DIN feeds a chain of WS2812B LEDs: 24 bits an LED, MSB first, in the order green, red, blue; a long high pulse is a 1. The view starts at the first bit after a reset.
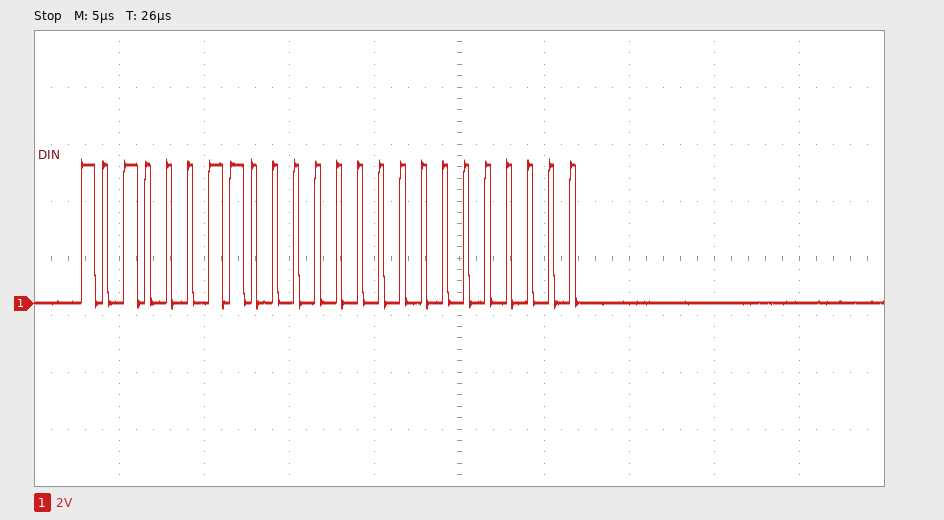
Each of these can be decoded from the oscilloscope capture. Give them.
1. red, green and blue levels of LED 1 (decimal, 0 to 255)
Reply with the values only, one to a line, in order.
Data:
0, 163, 0
